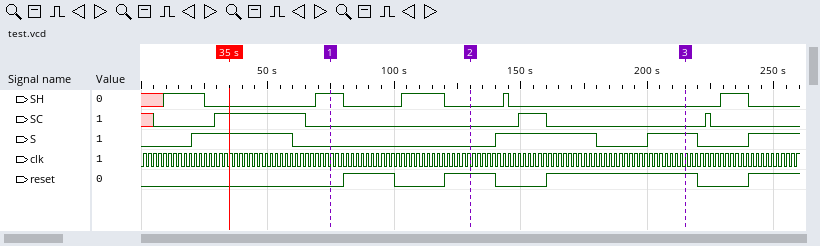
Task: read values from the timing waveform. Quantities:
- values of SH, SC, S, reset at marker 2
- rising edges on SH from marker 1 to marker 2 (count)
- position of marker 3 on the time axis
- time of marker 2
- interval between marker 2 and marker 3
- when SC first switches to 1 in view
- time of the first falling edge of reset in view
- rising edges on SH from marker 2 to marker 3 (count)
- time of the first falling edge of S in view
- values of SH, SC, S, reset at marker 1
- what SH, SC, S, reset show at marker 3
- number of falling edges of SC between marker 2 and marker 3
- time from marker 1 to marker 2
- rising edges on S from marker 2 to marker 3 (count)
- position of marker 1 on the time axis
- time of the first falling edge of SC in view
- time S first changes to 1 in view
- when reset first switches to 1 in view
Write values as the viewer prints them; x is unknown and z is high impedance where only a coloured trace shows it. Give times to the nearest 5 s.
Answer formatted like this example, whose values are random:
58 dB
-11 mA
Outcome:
SH=0, SC=0, S=0, reset=1
1
215 s
130 s
85 s
30 s
100 s
1
60 s
SH=1, SC=0, S=0, reset=0
SH=0, SC=0, S=1, reset=1
1
55 s
2
75 s
65 s
20 s
80 s
